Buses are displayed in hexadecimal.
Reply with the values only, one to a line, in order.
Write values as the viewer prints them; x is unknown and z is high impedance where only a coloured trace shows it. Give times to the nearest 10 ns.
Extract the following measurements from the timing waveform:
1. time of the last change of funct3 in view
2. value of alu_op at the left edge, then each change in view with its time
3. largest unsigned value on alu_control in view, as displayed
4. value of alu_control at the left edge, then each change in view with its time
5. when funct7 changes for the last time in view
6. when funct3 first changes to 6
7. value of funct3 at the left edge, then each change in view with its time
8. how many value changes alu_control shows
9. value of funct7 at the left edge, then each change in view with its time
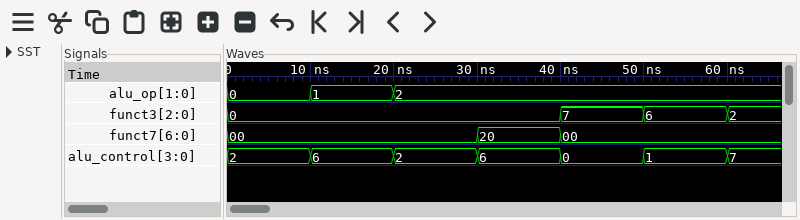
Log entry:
60 ns
0, 1 at 10 ns, 2 at 20 ns
7
2, 6 at 10 ns, 2 at 20 ns, 6 at 30 ns, 0 at 40 ns, 1 at 50 ns, 7 at 60 ns
40 ns
50 ns
0, 7 at 40 ns, 6 at 50 ns, 2 at 60 ns
6
00, 20 at 30 ns, 00 at 40 ns
